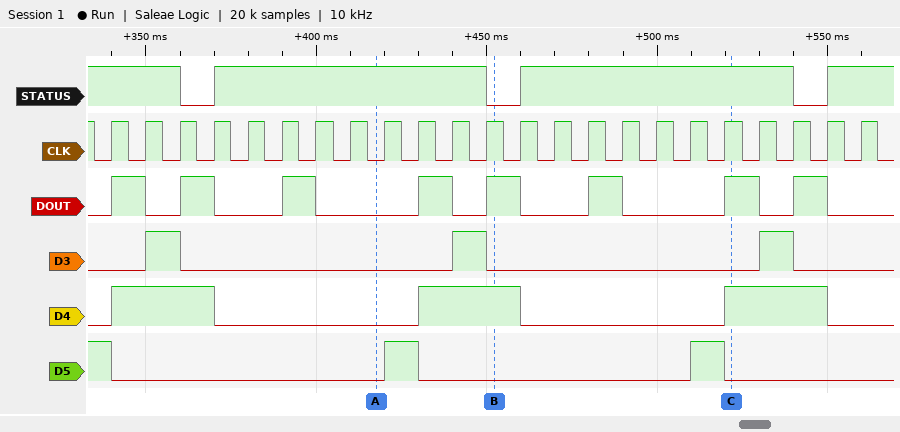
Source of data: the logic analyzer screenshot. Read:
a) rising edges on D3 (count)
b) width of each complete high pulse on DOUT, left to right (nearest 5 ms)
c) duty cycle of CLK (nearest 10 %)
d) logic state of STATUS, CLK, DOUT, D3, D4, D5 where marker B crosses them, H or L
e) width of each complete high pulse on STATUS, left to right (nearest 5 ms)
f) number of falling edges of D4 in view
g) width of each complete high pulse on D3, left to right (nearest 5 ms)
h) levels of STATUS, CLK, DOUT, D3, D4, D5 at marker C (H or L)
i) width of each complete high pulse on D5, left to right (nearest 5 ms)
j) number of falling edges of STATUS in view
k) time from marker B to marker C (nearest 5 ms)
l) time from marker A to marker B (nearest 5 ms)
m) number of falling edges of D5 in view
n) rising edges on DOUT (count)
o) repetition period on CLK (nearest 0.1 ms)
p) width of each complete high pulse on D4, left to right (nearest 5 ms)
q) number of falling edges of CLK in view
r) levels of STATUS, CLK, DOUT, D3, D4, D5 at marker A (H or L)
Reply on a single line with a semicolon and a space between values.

3; 10 ms, 10 ms, 10 ms, 10 ms, 10 ms, 10 ms, 10 ms, 10 ms; 50 %; STATUS=L, CLK=H, DOUT=H, D3=L, D4=H, D5=L; 80 ms, 80 ms; 3; 10 ms, 10 ms, 10 ms; STATUS=H, CLK=H, DOUT=H, D3=L, D4=H, D5=L; 10 ms, 10 ms; 3; 70 ms; 35 ms; 3; 8; 10 ms; 30 ms, 30 ms, 30 ms; 24; STATUS=H, CLK=L, DOUT=L, D3=L, D4=L, D5=L
